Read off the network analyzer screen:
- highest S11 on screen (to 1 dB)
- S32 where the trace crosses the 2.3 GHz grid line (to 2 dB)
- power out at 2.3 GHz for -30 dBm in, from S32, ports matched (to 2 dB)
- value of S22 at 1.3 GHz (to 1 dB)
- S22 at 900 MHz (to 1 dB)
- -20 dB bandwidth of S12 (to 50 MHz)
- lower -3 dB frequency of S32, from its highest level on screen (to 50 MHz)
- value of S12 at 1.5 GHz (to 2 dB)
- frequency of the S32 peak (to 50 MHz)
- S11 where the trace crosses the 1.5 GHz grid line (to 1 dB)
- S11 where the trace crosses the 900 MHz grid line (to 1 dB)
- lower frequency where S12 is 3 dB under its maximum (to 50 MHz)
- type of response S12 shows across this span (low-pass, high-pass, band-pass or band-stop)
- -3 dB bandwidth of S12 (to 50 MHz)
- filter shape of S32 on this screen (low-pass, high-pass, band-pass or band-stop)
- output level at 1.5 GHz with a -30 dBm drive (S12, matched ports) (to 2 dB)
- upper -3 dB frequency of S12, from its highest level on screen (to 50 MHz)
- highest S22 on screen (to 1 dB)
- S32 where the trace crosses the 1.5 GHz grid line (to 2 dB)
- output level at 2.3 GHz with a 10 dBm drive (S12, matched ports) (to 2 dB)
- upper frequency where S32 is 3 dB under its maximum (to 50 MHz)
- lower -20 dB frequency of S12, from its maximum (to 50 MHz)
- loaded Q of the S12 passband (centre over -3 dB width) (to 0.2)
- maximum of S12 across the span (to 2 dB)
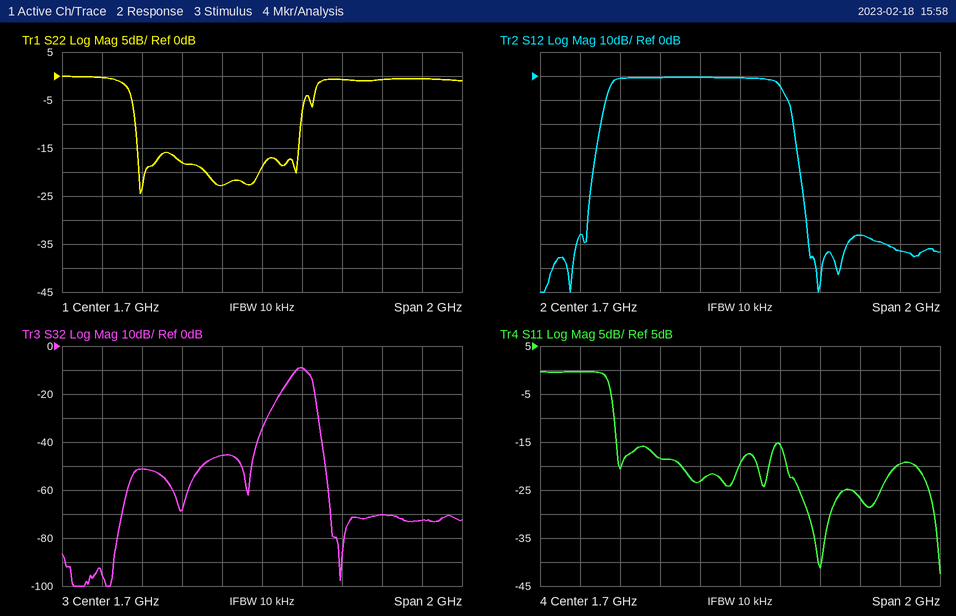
0 dB
-70 dB
-100 dBm
-18 dB
0 dB
950 MHz
1.85 GHz
0 dB
1.90 GHz
-23 dB
0 dB
1.05 GHz
band-pass
850 MHz
band-pass
-30 dBm
1.90 GHz
0 dB
-46 dB
-56 dBm
1.95 GHz
1.00 GHz
1.8
0 dB
